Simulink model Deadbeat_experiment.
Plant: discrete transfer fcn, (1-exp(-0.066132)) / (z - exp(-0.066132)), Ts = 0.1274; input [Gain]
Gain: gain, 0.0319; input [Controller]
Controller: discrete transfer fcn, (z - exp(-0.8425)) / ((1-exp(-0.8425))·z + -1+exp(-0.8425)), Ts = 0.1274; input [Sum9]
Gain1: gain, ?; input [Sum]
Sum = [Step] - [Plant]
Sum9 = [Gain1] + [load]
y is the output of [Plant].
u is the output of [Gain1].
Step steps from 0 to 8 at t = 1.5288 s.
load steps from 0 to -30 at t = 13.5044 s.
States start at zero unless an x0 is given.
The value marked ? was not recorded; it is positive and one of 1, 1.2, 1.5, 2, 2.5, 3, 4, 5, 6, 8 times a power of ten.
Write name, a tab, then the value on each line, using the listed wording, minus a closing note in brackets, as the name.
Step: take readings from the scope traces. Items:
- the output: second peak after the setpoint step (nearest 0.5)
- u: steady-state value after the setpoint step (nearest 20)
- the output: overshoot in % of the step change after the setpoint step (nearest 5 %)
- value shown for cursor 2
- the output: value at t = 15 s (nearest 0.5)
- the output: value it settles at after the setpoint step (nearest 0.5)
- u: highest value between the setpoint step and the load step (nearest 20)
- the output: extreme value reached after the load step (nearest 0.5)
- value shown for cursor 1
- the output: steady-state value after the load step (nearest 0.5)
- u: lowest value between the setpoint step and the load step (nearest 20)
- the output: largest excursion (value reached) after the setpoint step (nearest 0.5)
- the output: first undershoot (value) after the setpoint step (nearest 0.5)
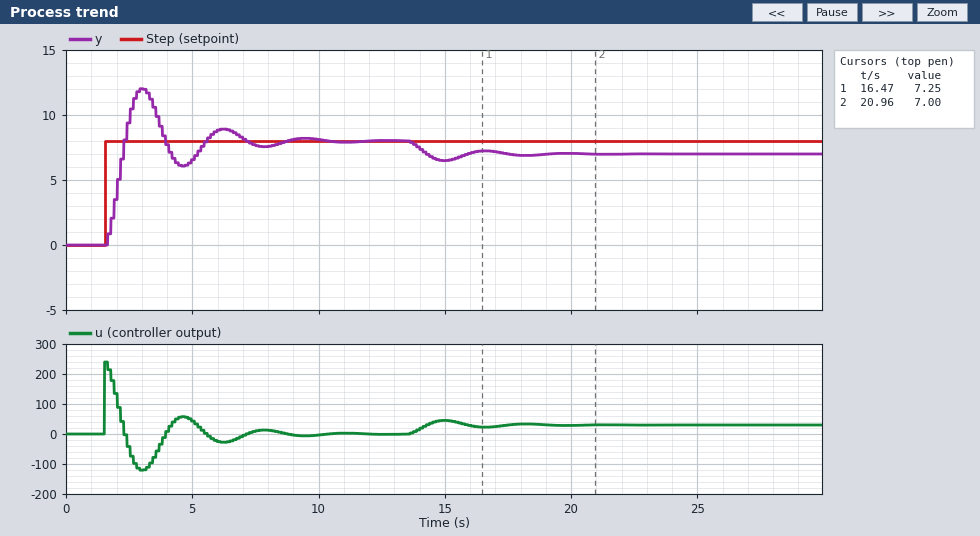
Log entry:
the output: second peak after the setpoint step	9.0
u: steady-state value after the setpoint step	0
the output: overshoot in % of the step change after the setpoint step	50 %
value shown for cursor 2	7.00
the output: value at t = 15 s	6.5
the output: value it settles at after the setpoint step	8.0
u: highest value between the setpoint step and the load step	240
the output: extreme value reached after the load step	6.5
value shown for cursor 1	7.25
the output: steady-state value after the load step	7.0
u: lowest value between the setpoint step and the load step	-120
the output: largest excursion (value reached) after the setpoint step	12.0
the output: first undershoot (value) after the setpoint step	6.0
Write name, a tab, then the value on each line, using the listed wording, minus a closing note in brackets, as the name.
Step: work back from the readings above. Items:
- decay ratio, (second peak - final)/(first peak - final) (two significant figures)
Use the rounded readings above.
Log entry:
decay ratio, (second peak - final)/(first peak - final)	0.25
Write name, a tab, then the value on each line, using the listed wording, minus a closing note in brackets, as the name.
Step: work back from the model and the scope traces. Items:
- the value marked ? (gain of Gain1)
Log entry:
the value marked ?	30
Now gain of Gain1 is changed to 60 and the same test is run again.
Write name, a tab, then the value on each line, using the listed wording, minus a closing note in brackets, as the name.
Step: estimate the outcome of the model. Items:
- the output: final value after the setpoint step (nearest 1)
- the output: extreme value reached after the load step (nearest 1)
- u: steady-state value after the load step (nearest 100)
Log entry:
the output: final value after the setpoint step	8
the output: extreme value reached after the load step	7
u: steady-state value after the load step	0
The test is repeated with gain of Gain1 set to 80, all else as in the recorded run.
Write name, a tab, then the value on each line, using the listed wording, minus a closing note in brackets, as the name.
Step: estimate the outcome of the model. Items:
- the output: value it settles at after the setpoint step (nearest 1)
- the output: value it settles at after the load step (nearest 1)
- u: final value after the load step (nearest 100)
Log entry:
the output: value it settles at after the setpoint step	8
the output: value it settles at after the load step	8
u: final value after the load step	0
